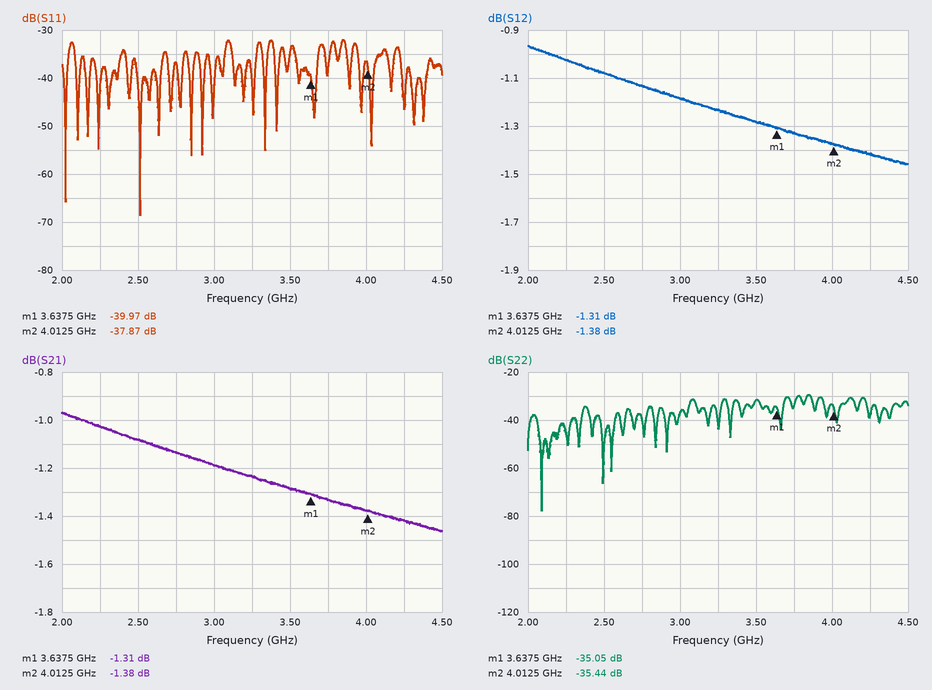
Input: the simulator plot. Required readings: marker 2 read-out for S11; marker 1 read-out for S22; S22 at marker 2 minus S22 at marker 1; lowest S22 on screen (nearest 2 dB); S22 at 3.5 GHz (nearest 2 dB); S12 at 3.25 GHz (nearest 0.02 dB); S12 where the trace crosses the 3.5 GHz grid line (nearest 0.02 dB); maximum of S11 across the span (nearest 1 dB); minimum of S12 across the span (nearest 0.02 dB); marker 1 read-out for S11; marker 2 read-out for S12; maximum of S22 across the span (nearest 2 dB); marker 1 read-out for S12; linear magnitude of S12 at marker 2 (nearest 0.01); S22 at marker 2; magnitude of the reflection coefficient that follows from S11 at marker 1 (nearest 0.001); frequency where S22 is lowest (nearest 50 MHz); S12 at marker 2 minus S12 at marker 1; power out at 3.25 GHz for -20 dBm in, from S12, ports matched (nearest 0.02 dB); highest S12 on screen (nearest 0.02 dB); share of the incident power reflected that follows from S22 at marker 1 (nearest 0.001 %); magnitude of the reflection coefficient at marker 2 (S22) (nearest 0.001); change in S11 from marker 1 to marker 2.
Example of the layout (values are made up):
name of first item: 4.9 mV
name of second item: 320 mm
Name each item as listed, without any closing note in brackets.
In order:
marker 2 read-out for S11: -37.87 dB
marker 1 read-out for S22: -35.05 dB
S22 at marker 2 minus S22 at marker 1: -0.39 dB
lowest S22 on screen: -78 dB
S22 at 3.5 GHz: -32 dB
S12 at 3.25 GHz: -1.24 dB
S12 where the trace crosses the 3.5 GHz grid line: -1.28 dB
maximum of S11 across the span: -32 dB
minimum of S12 across the span: -1.46 dB
marker 1 read-out for S11: -39.97 dB
marker 2 read-out for S12: -1.38 dB
maximum of S22 across the span: -30 dB
marker 1 read-out for S12: -1.31 dB
linear magnitude of S12 at marker 2: 0.85
S22 at marker 2: -35.44 dB
magnitude of the reflection coefficient that follows from S11 at marker 1: 0.010
frequency where S22 is lowest: 2.10 GHz
S12 at marker 2 minus S12 at marker 1: -0.07 dB
power out at 3.25 GHz for -20 dBm in, from S12, ports matched: -21.24 dBm
highest S12 on screen: -0.96 dB
share of the incident power reflected that follows from S22 at marker 1: 0.031 %
magnitude of the reflection coefficient at marker 2 (S22): 0.017
change in S11 from marker 1 to marker 2: 2.10 dB
